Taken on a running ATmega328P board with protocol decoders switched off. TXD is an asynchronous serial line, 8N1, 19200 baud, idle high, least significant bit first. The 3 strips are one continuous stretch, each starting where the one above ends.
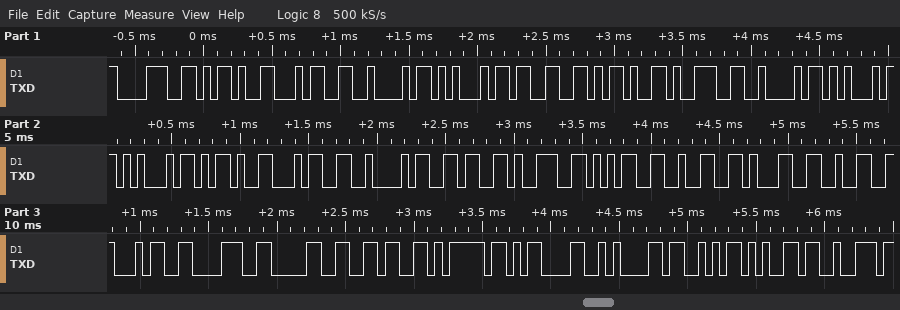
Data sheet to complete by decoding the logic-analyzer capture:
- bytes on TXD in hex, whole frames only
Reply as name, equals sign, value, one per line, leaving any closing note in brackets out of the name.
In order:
bytes on TXD in hex, whole frames only = 38 2D 34 42 45 33 2D 39 42 45 45 2D 34 42 36 39 35 32 31 32 34 38 30 36 7D 0D 0A 53 65 72
